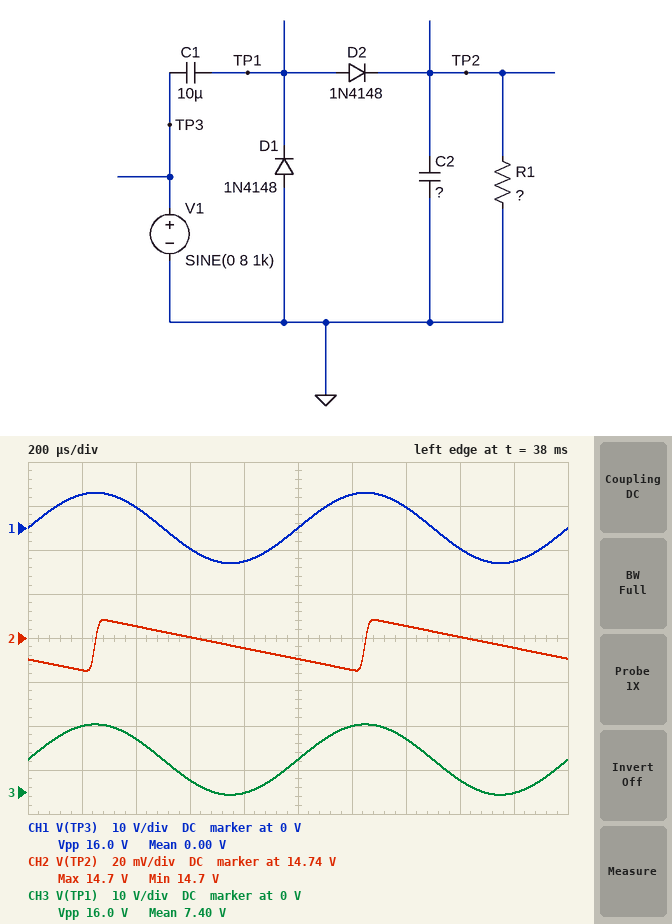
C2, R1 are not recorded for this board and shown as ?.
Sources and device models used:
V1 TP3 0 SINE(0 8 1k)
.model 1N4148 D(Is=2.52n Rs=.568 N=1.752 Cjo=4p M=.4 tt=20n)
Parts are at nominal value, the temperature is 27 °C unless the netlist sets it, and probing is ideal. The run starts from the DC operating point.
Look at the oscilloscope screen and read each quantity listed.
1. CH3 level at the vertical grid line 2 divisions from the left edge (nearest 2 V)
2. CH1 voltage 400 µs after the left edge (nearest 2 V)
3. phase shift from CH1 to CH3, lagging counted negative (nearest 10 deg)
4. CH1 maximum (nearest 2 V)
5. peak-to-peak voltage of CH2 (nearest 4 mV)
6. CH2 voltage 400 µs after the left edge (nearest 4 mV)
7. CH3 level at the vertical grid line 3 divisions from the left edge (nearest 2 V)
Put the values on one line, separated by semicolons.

12 V; 4 V; 0 deg; 8 V; 24 mV; 14.744 V; 2 V
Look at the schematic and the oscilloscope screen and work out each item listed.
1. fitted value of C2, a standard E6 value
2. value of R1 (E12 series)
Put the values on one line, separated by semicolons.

3.3 µF; 180 kΩ
